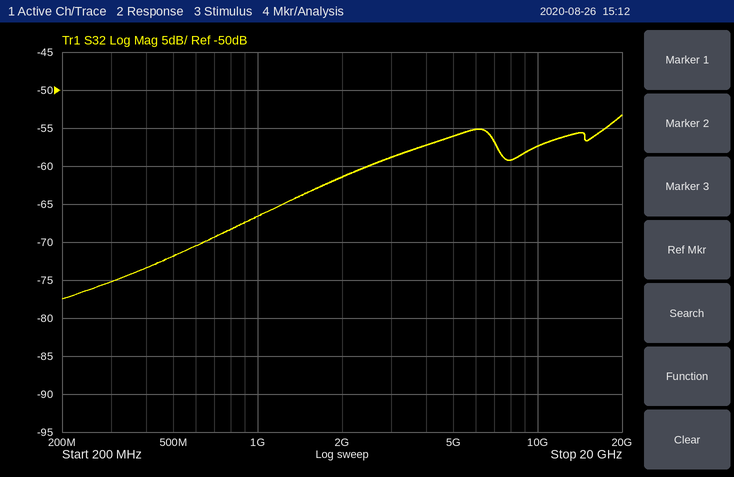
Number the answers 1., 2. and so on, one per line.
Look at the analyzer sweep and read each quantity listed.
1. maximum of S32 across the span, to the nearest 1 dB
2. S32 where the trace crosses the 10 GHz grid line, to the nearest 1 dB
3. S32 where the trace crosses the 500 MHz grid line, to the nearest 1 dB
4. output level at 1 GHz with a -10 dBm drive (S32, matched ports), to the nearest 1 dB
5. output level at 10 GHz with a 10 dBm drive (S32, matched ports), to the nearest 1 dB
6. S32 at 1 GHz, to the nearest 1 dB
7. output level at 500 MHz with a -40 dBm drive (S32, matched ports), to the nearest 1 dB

1. -53 dB
2. -57 dB
3. -72 dB
4. -77 dBm
5. -47 dBm
6. -67 dB
7. -112 dBm
